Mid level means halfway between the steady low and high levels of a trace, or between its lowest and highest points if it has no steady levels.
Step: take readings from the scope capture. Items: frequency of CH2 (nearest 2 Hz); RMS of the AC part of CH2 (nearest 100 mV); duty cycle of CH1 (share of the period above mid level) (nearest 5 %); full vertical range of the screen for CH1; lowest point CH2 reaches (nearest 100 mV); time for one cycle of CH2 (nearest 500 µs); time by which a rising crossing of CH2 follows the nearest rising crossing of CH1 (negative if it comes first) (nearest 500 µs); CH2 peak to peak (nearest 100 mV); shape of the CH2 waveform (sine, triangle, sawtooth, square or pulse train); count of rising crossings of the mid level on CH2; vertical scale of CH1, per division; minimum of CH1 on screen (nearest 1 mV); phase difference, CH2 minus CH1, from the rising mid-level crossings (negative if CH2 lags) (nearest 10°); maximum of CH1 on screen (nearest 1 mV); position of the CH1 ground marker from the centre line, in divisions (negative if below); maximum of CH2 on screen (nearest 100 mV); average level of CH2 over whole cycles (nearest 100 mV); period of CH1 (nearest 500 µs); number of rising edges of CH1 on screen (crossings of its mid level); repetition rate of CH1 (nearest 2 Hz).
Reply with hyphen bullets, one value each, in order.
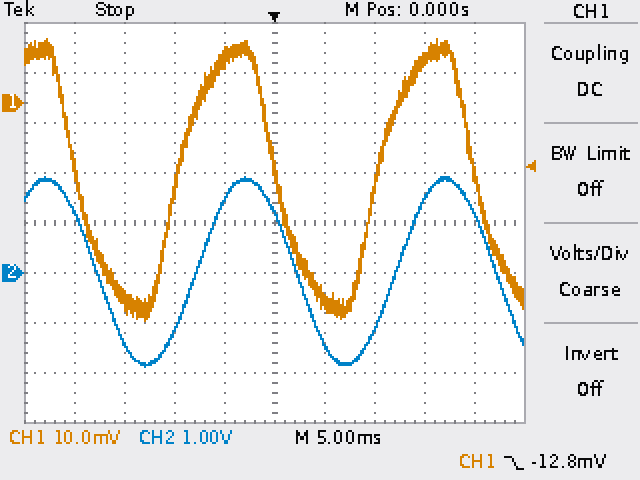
- 50 Hz
- 1.3 V
- 50 %
- 80 mV
- -1.9 V
- 20.0 ms
- +2.0 ms
- 3.8 V
- sine
- 2
- 10 mV
- -44 mV
- -40°
- 13 mV
- +2.4 div
- 1.9 V
- 0.0 V
- 20.0 ms
- 2
- 50 Hz
